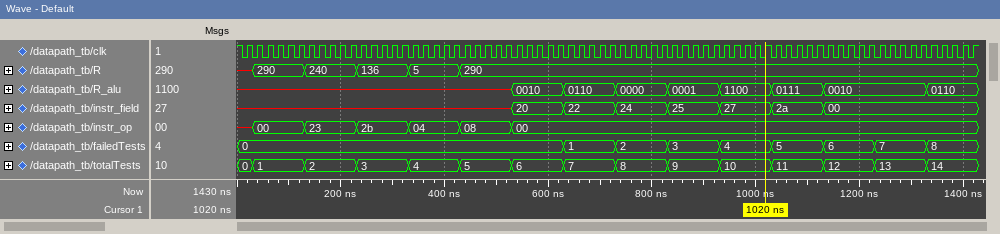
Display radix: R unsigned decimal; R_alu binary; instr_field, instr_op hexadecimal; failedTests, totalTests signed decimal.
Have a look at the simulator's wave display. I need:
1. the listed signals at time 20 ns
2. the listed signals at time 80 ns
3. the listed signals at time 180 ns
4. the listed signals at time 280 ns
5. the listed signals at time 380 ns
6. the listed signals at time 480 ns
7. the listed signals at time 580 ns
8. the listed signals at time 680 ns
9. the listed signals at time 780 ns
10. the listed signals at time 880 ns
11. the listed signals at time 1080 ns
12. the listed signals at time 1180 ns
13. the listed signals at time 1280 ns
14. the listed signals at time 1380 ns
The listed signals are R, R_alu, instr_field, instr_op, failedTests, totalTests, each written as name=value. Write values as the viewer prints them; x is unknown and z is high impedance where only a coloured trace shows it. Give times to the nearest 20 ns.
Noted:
R=x, R_alu=x, instr_field=x, instr_op=x, failedTests=0, totalTests=0
R=290, R_alu=x, instr_field=x, instr_op=00, failedTests=0, totalTests=1
R=240, R_alu=x, instr_field=x, instr_op=23, failedTests=0, totalTests=2
R=136, R_alu=x, instr_field=x, instr_op=2b, failedTests=0, totalTests=3
R=5, R_alu=x, instr_field=x, instr_op=04, failedTests=0, totalTests=4
R=290, R_alu=x, instr_field=x, instr_op=08, failedTests=0, totalTests=5
R=290, R_alu=0010, instr_field=20, instr_op=00, failedTests=0, totalTests=6
R=290, R_alu=0110, instr_field=22, instr_op=00, failedTests=1, totalTests=7
R=290, R_alu=0000, instr_field=24, instr_op=00, failedTests=2, totalTests=8
R=290, R_alu=0001, instr_field=25, instr_op=00, failedTests=3, totalTests=9
R=290, R_alu=0111, instr_field=2a, instr_op=00, failedTests=5, totalTests=11
R=290, R_alu=0010, instr_field=00, instr_op=00, failedTests=6, totalTests=12
R=290, R_alu=0010, instr_field=00, instr_op=00, failedTests=7, totalTests=13
R=290, R_alu=0110, instr_field=00, instr_op=00, failedTests=8, totalTests=14
